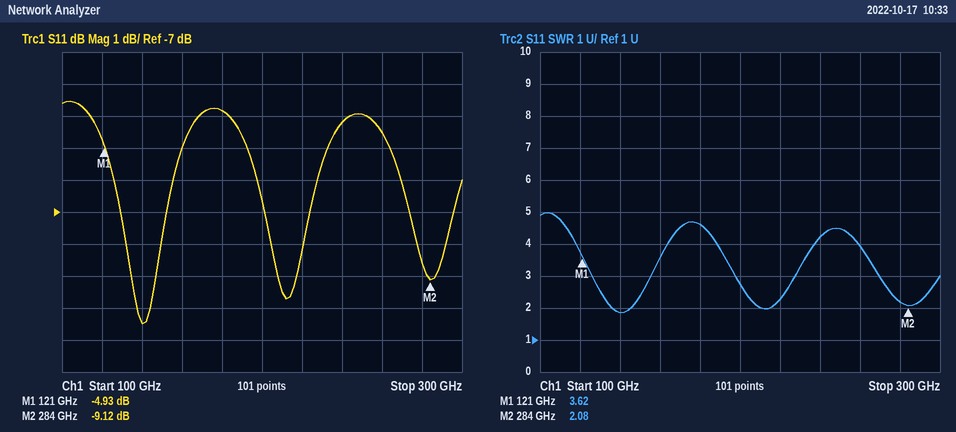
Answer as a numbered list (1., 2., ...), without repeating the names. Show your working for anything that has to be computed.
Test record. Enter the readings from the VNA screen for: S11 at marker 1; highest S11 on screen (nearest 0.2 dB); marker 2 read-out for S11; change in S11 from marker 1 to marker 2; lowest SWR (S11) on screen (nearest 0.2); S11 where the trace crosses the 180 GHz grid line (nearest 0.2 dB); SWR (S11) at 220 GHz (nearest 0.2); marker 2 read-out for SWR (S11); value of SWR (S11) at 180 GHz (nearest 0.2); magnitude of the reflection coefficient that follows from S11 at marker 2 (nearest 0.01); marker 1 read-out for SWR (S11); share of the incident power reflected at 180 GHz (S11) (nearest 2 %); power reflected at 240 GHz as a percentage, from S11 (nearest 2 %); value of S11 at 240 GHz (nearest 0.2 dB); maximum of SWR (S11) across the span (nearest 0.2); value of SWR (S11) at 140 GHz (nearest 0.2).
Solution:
1. -4.93 dB
2. -3.6 dB
3. -9.12 dB
4. -9.12 − (-4.93) = -4.19 dB
5. 1.8
6. -3.8 dB
7. 2.2
8. 2.08
9. 4.6
10. 10^(-9.12/20) ≈ 0.35
11. 3.62
12. 10^(-3.8/10) ≈ 42 %
13. 10^(-4.2/10) ≈ 38 %
14. -4.2 dB
15. 5.0
16. 1.8
